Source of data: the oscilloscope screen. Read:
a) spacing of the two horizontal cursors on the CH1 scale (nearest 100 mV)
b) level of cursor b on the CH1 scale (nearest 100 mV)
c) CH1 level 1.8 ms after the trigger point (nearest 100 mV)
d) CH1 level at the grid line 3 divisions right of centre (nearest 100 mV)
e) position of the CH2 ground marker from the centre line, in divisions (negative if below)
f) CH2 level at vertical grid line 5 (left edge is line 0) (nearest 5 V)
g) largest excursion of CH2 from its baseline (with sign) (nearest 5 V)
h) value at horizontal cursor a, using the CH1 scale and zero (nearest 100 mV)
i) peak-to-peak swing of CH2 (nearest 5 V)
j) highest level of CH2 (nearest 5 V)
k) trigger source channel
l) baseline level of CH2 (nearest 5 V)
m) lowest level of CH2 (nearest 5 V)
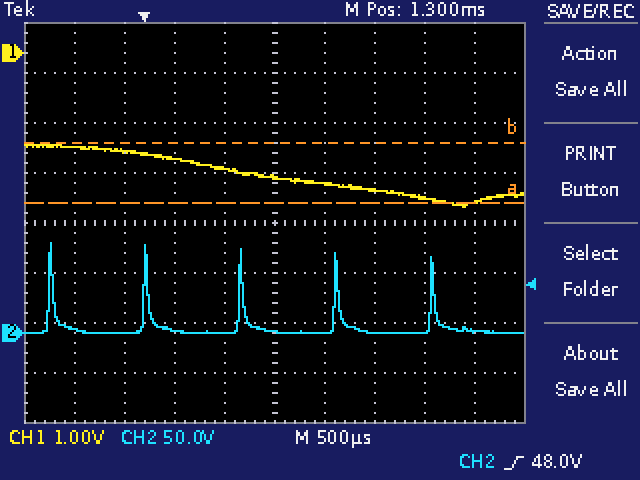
1.2 V
-1.8 V
-2.6 V
-2.9 V
-2.2 div
0 V
+90 V
-3.0 V
90 V
90 V
CH2
0 V
0 V
